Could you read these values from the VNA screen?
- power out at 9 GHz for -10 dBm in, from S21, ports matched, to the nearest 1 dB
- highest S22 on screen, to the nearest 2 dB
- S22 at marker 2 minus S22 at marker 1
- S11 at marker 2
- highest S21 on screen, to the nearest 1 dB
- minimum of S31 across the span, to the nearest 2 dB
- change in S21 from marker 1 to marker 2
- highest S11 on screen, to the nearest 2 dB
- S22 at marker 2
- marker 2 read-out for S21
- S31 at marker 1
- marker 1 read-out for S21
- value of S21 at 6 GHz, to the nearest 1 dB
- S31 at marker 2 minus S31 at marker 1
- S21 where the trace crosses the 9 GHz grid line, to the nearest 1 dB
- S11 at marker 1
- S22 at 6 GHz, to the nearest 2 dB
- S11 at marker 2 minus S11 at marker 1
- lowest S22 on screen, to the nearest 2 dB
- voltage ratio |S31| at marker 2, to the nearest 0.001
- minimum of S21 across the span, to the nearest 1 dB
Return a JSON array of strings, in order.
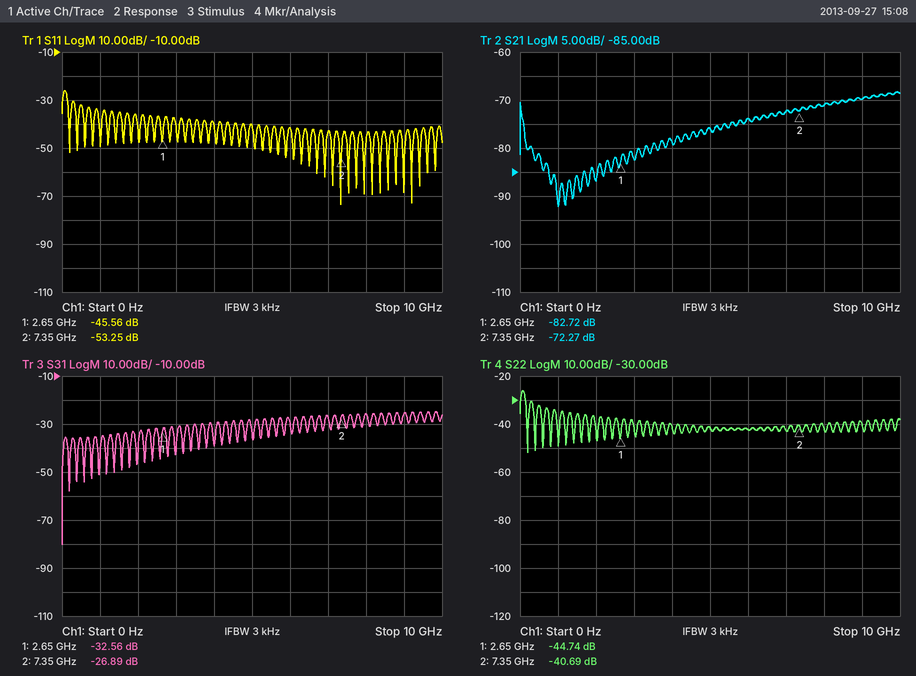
["-80 dBm", "-26 dB", "4.05 dB", "-53.25 dB", "-68 dB", "-80 dB", "10.45 dB", "-26 dB", "-40.69 dB", "-72.27 dB", "-32.56 dB", "-82.72 dB", "-74 dB", "5.67 dB", "-70 dB", "-45.56 dB", "-42 dB", "-7.69 dB", "-52 dB", "0.045", "-92 dB"]
